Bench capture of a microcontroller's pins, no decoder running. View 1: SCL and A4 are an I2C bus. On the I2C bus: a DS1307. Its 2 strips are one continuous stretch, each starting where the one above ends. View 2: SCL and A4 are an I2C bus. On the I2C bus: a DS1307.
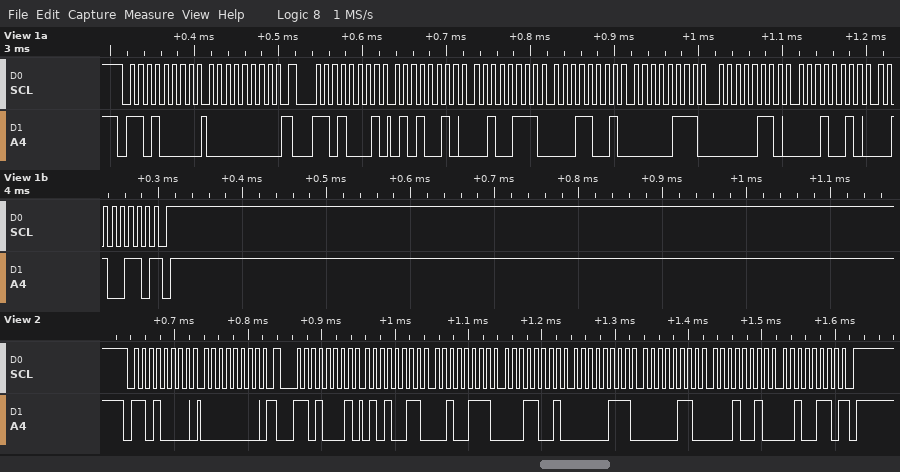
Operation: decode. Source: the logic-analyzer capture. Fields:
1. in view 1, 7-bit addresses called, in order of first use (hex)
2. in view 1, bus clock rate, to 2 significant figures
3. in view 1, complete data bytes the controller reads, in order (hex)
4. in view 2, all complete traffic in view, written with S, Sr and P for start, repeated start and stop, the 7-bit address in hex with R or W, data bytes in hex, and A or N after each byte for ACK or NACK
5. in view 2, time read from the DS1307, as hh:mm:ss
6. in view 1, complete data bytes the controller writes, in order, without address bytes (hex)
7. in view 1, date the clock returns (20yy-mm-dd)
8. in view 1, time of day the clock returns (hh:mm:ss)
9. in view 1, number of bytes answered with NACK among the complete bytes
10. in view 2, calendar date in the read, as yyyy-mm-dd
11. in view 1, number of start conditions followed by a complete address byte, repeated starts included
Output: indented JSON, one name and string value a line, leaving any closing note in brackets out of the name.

{
  "in view 1, 7-bit addresses called, in order of first use": "0x68",
  "in view 1, bus clock rate, to 2 significant figures": "100 kHz",
  "in view 1, complete data bytes the controller reads, in order": "52 27 19 07 06 12 26",
  "in view 2, all complete traffic in view, written with S, Sr and P for start, repeated start and stop, the 7-bit address in hex with R or W, data bytes in hex, and A or N after each byte for ACK or NACK": "S 68W A 00 A Sr 68R A 53 A 27 A 19 A 07 A 06 A 12 A 26 N P",
  "in view 2, time read from the DS1307, as hh:mm:ss": "19:27:53",
  "in view 1, complete data bytes the controller writes, in order, without address bytes": "00",
  "in view 1, date the clock returns": "2026-12-06",
  "in view 1, time of day the clock returns": "19:27:52",
  "in view 1, number of bytes answered with NACK among the complete bytes": "1",
  "in view 2, calendar date in the read, as yyyy-mm-dd": "2026-12-06",
  "in view 1, number of start conditions followed by a complete address byte, repeated starts included": "2"
}
